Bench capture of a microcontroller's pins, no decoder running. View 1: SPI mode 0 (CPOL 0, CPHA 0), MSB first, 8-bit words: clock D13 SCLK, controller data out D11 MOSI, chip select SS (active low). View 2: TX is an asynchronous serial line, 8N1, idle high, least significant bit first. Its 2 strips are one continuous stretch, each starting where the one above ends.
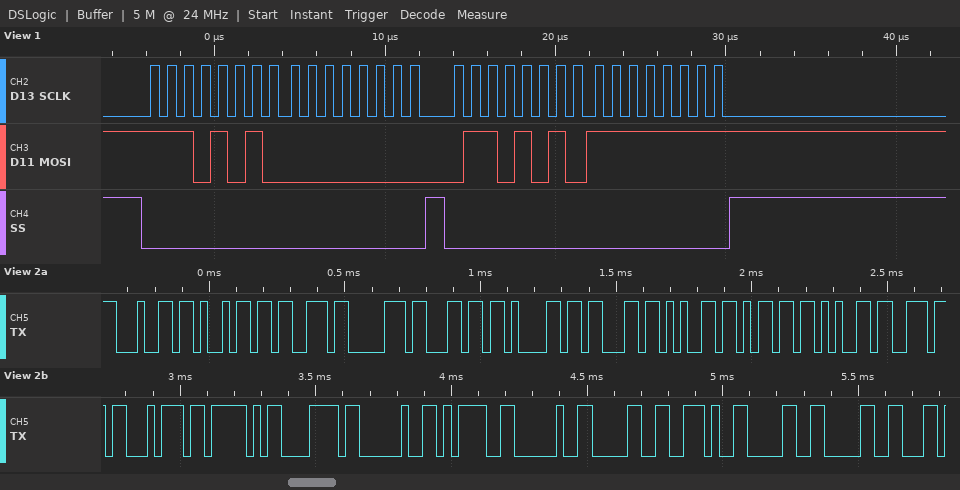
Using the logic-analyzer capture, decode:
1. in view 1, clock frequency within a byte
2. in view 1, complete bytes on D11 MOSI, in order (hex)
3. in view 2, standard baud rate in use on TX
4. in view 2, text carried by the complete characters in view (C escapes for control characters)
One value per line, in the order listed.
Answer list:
1 MHz
0xEA 0x00 0x6A 0xFF
38400 baud
"displacement_x = 0.00"
